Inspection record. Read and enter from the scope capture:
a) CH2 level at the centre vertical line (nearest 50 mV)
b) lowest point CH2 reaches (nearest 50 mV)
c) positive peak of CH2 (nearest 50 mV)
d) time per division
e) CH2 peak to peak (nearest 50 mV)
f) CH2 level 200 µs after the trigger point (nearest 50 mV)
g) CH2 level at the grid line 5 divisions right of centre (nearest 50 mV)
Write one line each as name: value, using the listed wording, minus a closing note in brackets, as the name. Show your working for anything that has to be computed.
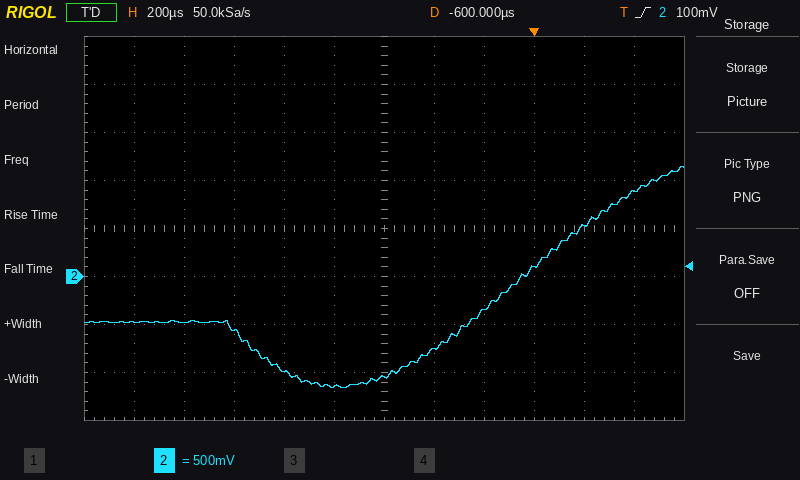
CH2 level at the centre vertical line: -1.05 V
lowest point CH2 reaches: -1.15 V
positive peak of CH2: 1.15 V
time per division: 200 µs
CH2 peak to peak: 1.15 V − (-1.15 V) = 2.30 V
CH2 level 200 µs after the trigger point: 550 mV
CH2 level at the grid line 5 divisions right of centre: 900 mV
